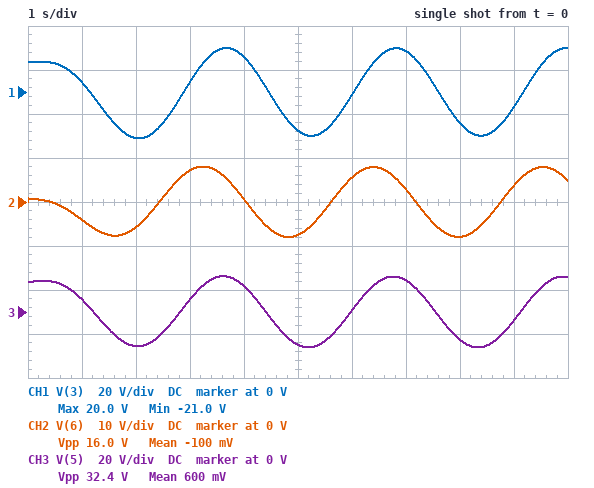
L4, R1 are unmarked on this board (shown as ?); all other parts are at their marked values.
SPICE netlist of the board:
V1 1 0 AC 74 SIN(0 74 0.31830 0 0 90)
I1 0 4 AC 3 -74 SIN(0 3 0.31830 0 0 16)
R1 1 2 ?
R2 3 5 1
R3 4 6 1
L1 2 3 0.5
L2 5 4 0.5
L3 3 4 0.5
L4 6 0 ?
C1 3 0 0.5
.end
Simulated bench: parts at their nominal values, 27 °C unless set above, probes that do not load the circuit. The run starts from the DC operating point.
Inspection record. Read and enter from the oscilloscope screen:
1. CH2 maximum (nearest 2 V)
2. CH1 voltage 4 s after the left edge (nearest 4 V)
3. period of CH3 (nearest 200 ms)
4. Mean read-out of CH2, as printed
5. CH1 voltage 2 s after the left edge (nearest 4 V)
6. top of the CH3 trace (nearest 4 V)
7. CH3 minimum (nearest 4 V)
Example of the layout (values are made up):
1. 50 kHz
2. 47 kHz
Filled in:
1. 8 V
2. 16 V
3. 3.2 s
4. -100 mV
5. -20 V
6. 16 V
7. -16 V
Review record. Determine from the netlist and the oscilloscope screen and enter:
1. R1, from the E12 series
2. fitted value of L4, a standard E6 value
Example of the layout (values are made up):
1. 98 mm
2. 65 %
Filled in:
1. 4.7 Ω
2. 330 mH
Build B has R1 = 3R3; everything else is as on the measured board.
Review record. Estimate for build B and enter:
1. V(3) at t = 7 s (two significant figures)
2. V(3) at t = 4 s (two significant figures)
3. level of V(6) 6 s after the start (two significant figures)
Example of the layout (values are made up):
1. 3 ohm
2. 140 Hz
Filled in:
1. 24 V
2. 20 V
3. 7.5 V
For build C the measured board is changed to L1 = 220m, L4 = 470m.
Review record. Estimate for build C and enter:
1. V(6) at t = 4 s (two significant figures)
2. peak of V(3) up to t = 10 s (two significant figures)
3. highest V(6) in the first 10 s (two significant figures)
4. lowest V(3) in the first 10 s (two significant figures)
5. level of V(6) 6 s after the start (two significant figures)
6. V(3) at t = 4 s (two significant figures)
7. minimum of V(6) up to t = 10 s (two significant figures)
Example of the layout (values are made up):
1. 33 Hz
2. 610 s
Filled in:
1. 1.8 V
2. 21 V
3. 11 V
4. -23 V
5. 6.7 V
6. 17 V
7. -11 V
